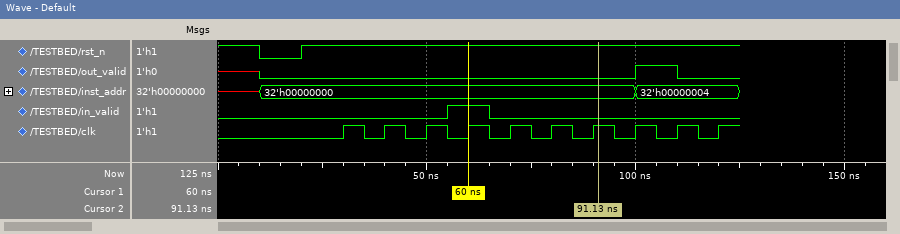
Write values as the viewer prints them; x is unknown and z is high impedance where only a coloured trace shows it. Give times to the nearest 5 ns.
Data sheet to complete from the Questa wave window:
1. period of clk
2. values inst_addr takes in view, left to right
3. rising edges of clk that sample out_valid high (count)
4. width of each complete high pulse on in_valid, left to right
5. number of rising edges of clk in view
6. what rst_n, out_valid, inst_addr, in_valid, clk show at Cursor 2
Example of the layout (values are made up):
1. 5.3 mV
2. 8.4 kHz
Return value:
1. 10 ns
2. x, 32'h00000000, 32'h00000004
3. 1
4. 10 ns
5. 10
6. rst_n=1, out_valid=0, inst_addr=32'h00000000, in_valid=0, clk=1
